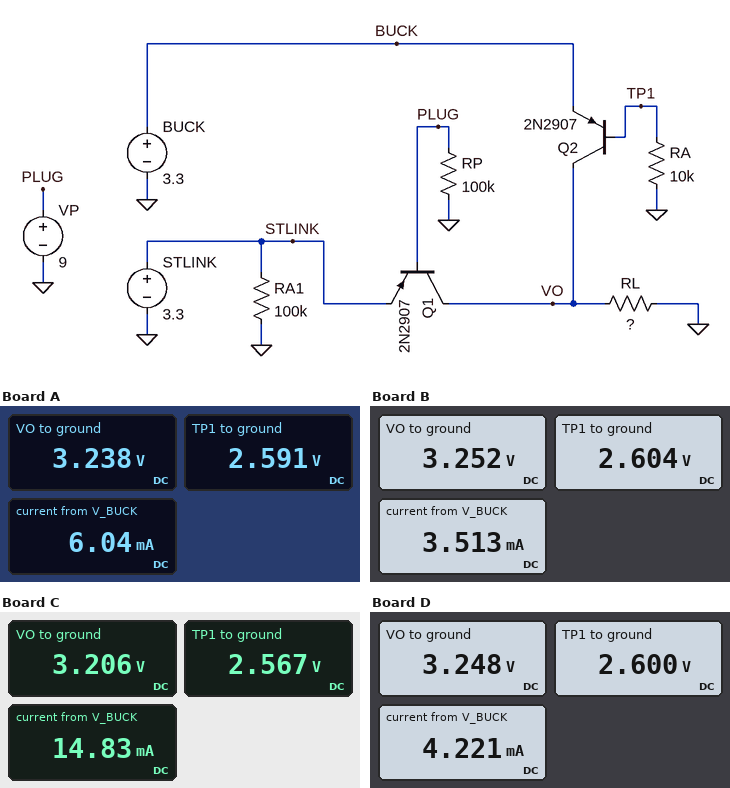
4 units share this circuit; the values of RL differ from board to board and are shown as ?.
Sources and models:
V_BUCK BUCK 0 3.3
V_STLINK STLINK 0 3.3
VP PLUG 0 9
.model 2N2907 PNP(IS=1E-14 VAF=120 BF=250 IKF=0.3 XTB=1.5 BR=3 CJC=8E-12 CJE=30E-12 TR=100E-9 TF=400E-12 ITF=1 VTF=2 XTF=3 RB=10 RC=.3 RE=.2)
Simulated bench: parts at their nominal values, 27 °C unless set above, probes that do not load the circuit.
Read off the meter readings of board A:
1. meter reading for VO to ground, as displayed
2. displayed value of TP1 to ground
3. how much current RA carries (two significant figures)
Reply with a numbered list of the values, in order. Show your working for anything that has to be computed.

1. 3.238 V
2. 2.591 V
3. (2.591 V) / 10 kΩ = 260 µA
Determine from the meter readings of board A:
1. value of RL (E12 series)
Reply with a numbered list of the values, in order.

1. 560 Ω
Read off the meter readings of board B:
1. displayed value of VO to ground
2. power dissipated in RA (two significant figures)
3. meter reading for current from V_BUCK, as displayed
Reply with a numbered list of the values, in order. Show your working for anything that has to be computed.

1. 3.252 V
2. (2.604 V)^2 / 10 kΩ = 680 µW
3. 3.513 mA
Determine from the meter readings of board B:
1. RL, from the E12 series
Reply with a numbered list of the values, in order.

1. 1 kΩ
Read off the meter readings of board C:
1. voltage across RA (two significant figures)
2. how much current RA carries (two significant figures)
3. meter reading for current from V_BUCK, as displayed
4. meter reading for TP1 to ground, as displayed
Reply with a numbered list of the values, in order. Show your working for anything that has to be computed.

1. 2.567 V = 2.6 V
2. (2.567 V) / 10 kΩ = 260 µA
3. 14.83 mA
4. 2.567 V
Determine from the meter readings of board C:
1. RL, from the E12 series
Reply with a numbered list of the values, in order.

1. 220 Ω
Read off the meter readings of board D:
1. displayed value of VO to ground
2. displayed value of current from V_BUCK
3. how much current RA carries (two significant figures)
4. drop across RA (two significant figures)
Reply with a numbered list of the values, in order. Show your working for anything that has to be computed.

1. 3.248 V
2. 4.221 mA
3. (2.6 V) / 10 kΩ = 260 µA
4. 2.6 V = 2.6 V
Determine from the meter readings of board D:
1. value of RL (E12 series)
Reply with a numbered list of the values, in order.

1. 820 Ω
